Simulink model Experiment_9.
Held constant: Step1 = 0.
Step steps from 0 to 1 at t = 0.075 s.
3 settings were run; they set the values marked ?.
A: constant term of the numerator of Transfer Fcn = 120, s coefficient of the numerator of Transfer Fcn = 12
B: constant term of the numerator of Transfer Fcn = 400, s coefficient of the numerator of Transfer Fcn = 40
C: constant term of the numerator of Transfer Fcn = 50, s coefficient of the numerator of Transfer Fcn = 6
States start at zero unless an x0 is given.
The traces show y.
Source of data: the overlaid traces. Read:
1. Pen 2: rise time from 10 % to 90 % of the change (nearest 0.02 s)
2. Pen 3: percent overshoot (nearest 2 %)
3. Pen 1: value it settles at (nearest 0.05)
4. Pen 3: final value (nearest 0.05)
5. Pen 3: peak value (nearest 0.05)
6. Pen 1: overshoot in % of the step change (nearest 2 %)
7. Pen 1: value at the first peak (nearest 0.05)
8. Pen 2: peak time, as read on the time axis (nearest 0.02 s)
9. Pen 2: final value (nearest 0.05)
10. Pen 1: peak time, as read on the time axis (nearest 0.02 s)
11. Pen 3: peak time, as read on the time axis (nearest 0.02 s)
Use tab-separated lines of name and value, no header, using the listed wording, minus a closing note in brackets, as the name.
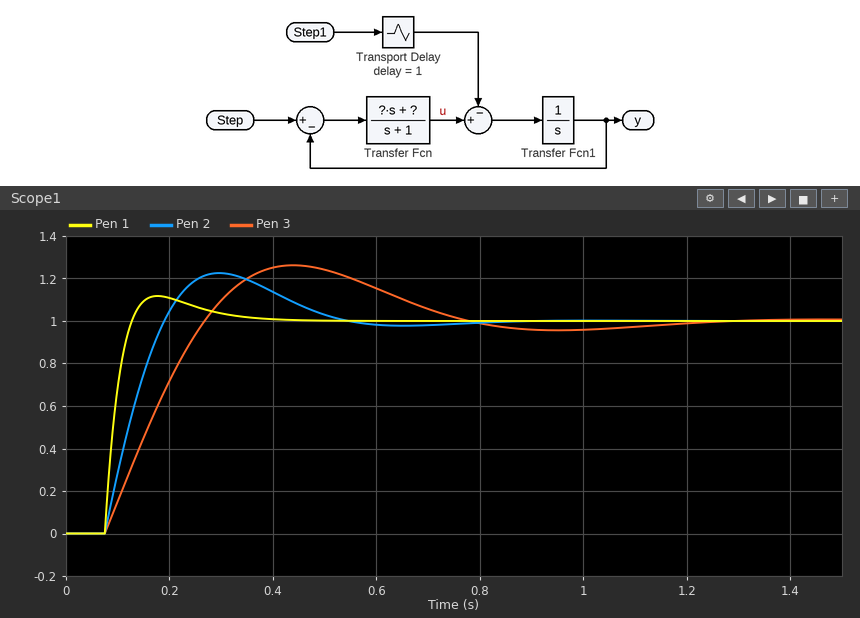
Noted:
Pen 2: rise time from 10 % to 90 % of the change	0.08 s
Pen 3: percent overshoot	26 %
Pen 1: value it settles at	1.00
Pen 3: final value	1.00
Pen 3: peak value	1.25
Pen 1: overshoot in % of the step change	12 %
Pen 1: value at the first peak	1.10
Pen 2: peak time, as read on the time axis	0.30 s
Pen 2: final value	1.00
Pen 1: peak time, as read on the time axis	0.18 s
Pen 3: peak time, as read on the time axis	0.44 s
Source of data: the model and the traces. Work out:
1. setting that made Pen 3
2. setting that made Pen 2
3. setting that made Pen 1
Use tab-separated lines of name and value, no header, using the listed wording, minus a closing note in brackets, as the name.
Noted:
setting that made Pen 3	C
setting that made Pen 2	A
setting that made Pen 1	B
